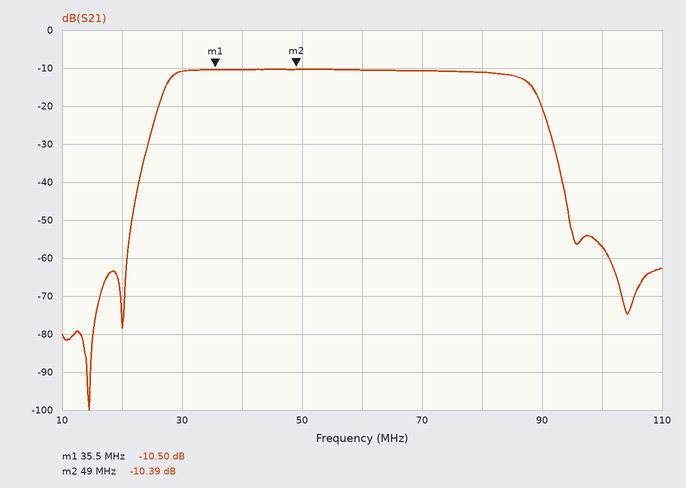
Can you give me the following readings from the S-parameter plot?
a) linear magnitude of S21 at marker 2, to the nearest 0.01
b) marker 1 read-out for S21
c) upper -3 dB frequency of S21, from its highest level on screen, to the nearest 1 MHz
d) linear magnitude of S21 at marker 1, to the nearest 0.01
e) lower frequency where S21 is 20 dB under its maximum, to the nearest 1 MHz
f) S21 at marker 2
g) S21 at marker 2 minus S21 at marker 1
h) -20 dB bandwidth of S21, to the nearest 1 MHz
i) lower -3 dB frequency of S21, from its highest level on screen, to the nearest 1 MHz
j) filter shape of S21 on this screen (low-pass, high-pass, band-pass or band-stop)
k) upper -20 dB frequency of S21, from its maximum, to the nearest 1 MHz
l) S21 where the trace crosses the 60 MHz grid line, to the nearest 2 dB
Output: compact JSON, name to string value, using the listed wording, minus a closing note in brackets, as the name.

{"linear magnitude of S21 at marker 2, to the nearest 0.01": "0.30", "marker 1 read-out for S21": "-10.50 dB", "upper -3 dB frequency of S21, from its highest level on screen, to the nearest 1 MHz": "87 MHz", "linear magnitude of S21 at marker 1, to the nearest 0.01": "0.30", "lower frequency where S21 is 20 dB under its maximum, to the nearest 1 MHz": "24 MHz", "S21 at marker 2": "-10.39 dB", "S21 at marker 2 minus S21 at marker 1": "0.11 dB", "-20 dB bandwidth of S21, to the nearest 1 MHz": "68 MHz", "lower -3 dB frequency of S21, from its highest level on screen, to the nearest 1 MHz": "28 MHz", "filter shape of S21 on this screen": "band-pass", "upper -20 dB frequency of S21, from its maximum, to the nearest 1 MHz": "92 MHz", "S21 where the trace crosses the 60 MHz grid line, to the nearest 2 dB": "-10 dB"}
